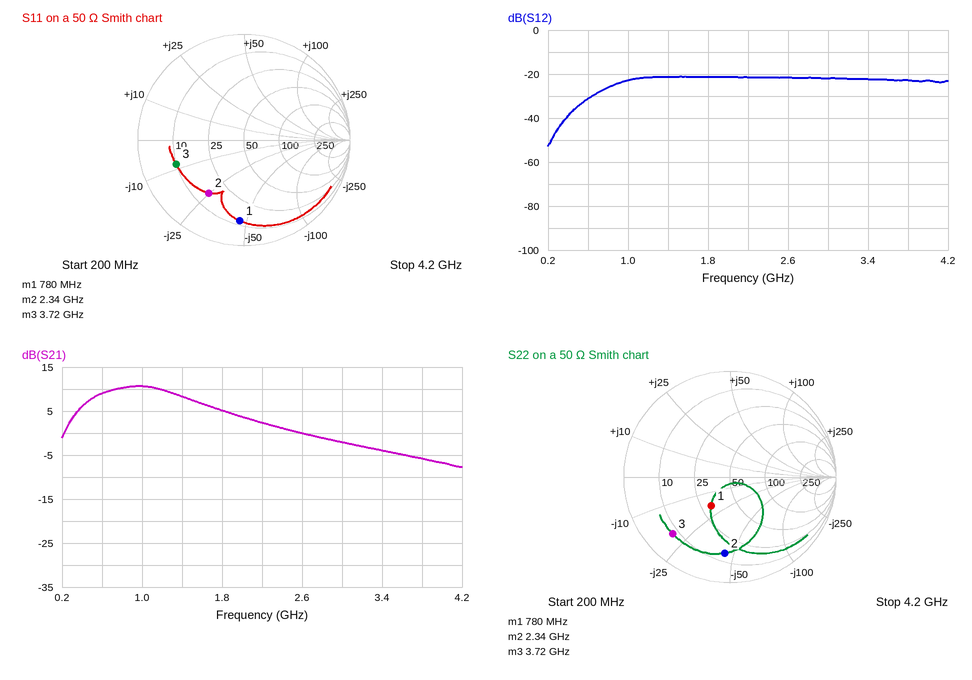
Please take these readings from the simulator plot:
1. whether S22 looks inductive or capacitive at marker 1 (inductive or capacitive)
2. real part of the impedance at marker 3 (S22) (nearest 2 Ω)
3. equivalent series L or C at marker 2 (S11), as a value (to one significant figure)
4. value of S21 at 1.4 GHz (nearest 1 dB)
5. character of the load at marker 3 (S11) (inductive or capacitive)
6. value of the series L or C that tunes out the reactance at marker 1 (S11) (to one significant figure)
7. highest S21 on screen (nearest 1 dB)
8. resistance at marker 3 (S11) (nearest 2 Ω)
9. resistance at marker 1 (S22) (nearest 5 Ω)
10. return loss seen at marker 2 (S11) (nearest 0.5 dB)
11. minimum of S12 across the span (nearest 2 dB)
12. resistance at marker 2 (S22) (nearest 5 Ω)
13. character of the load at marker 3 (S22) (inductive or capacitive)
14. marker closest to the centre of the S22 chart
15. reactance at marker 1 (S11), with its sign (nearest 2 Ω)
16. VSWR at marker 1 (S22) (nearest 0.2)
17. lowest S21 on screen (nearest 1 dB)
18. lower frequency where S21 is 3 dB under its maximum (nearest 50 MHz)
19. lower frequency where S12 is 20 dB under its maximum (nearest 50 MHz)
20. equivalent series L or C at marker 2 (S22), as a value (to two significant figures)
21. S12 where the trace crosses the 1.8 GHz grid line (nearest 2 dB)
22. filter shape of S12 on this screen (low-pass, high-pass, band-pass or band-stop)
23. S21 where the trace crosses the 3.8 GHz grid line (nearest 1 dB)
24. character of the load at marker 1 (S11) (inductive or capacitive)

capacitive
8 Ω
3 pF
8 dB
capacitive
9 nH
11 dB
10 Ω
30 Ω
4.5 dB
-52 dB
15 Ω
capacitive
marker 1
-46 Ω
2.0
-8 dB
500 MHz
350 MHz
1.5 pF
-22 dB
high-pass
-6 dB
capacitive
